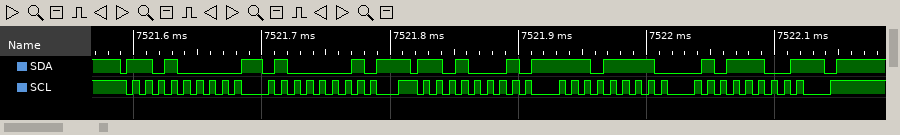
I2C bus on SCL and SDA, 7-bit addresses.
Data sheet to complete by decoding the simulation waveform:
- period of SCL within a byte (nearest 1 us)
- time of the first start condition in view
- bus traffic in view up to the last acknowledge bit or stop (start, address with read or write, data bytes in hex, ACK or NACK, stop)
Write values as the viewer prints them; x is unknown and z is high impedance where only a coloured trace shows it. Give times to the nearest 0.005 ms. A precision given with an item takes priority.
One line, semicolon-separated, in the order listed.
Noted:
10 us; 7521.59 ms; start, address 68 write ACK, 41 ACK, repeated start, address 68 read ACK, EF ACK, 5C NACK, stop
